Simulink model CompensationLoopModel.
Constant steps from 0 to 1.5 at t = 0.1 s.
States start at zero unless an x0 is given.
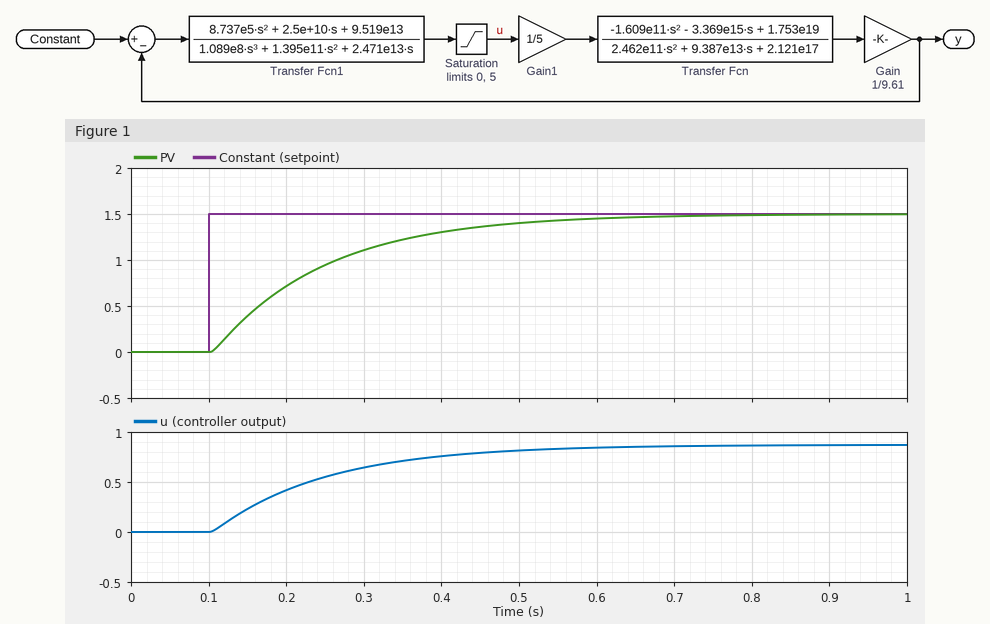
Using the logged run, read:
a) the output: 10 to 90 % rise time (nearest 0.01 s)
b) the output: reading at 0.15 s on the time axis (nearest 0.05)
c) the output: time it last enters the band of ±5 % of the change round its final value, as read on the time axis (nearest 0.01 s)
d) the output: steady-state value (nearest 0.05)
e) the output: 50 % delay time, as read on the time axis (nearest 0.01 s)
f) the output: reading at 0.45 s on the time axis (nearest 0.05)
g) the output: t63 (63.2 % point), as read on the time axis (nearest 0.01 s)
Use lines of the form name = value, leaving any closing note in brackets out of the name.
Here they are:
the output: 10 to 90 % rise time = 0.32 s
the output: reading at 0.15 s on the time axis = 0.40
the output: time it last enters the band of ±5 % of the change round its final value, as read on the time axis = 0.54 s
the output: steady-state value = 1.50
the output: 50 % delay time, as read on the time axis = 0.21 s
the output: reading at 0.45 s on the time axis = 1.35
the output: t63 (63.2 % point), as read on the time axis = 0.25 s
